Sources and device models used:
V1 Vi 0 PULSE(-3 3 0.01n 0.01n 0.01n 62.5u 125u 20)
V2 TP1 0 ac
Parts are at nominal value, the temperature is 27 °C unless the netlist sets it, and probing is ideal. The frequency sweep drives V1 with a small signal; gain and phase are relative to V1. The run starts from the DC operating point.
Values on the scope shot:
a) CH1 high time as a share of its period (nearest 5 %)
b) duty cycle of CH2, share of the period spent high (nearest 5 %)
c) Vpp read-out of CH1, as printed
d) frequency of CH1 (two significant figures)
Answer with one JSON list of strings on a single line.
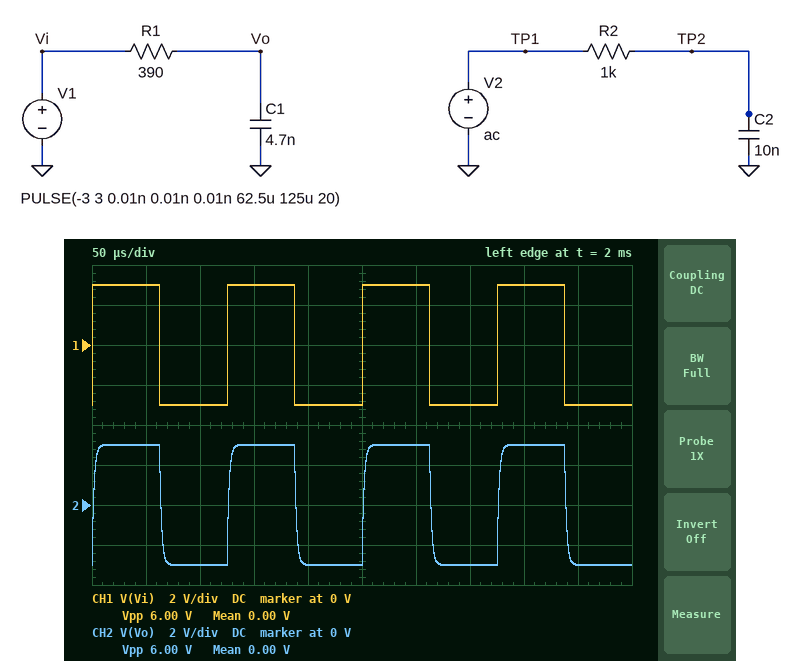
["50 %", "50 %", "6.00 V", "8.0 kHz"]
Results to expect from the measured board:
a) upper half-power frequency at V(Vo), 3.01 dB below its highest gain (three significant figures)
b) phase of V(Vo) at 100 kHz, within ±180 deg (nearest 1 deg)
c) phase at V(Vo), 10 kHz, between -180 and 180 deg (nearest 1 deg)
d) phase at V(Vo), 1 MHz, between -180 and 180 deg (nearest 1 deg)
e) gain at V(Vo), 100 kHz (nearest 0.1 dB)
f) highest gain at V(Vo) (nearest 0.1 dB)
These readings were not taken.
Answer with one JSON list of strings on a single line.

["86.8 kHz", "-49 deg", "-7 deg", "-85 deg", "-3.7 dB", "0 dB"]
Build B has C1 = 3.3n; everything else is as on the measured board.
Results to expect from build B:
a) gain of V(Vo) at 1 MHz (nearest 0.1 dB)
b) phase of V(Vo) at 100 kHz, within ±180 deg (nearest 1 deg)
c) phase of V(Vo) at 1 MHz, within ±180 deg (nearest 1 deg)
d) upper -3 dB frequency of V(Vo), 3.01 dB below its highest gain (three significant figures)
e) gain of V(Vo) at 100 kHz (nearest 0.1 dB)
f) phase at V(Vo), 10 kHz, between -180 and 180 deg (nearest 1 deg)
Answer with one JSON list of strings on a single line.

["-18.2 dB", "-39 deg", "-83 deg", "124 kHz", "-2.2 dB", "-5 deg"]
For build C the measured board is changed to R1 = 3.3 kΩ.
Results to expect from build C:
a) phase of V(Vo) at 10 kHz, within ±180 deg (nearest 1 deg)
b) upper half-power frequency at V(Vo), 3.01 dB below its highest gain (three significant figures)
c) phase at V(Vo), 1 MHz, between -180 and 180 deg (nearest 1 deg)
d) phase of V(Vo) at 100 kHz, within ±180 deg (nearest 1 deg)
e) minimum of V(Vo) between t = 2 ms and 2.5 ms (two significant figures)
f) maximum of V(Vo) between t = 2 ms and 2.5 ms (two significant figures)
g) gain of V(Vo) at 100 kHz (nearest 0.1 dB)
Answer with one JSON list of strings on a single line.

["-44 deg", "10.3 kHz", "-89 deg", "-84 deg", "-2.9 V", "2.9 V", "-19.8 dB"]
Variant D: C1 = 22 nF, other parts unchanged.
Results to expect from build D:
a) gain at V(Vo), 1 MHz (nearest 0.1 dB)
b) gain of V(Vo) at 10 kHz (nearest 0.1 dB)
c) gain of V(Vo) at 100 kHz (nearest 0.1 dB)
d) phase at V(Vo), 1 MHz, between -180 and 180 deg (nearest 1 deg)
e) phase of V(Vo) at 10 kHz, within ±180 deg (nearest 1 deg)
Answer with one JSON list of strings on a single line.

["-34.6 dB", "-1.1 dB", "-14.8 dB", "-89 deg", "-28 deg"]
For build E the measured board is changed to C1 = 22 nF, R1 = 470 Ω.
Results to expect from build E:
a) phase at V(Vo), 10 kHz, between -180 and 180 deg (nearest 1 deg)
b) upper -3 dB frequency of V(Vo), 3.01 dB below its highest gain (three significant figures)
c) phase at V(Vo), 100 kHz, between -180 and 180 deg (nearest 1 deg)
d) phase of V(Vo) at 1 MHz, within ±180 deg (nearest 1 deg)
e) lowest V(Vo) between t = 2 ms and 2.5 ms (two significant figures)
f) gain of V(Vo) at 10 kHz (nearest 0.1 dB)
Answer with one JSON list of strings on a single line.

["-33 deg", "15.4 kHz", "-81 deg", "-89 deg", "-3.0 V", "-1.5 dB"]
